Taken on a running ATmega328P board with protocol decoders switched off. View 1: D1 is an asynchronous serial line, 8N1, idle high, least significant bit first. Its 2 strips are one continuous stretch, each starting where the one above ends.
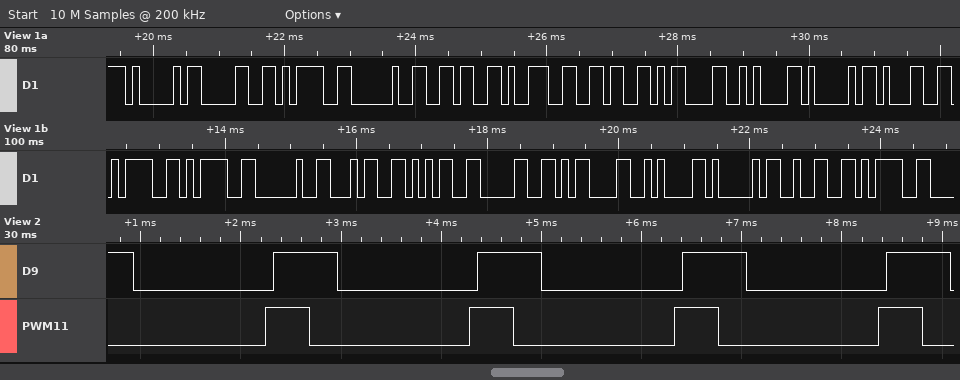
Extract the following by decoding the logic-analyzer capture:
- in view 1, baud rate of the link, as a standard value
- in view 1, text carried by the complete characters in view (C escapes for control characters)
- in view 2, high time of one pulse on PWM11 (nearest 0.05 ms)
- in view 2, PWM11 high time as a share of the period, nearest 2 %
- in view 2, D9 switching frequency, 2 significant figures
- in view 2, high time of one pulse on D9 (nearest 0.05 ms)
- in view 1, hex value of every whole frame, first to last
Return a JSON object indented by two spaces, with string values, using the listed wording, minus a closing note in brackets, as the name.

{
  "in view 1, baud rate of the link, as a standard value": "9600 baud",
  "in view 1, text carried by the complete characters in view": "\"A0= 696\\r\\nA1== 450\\r\\nA2=\"",
  "in view 2, high time of one pulse on PWM11": "0.45 ms",
  "in view 2, PWM11 high time as a share of the period, nearest 2 %": "22 %",
  "in view 2, D9 switching frequency, 2 significant figures": "490 Hz",
  "in view 2, high time of one pulse on D9": "0.65 ms",
  "in view 1, hex value of every whole frame, first to last": "41 30 3D 20 36 39 36 0D 0A 41 31 3D 3D 20 34 35 30 0D 0A 41 32 3D"
}
